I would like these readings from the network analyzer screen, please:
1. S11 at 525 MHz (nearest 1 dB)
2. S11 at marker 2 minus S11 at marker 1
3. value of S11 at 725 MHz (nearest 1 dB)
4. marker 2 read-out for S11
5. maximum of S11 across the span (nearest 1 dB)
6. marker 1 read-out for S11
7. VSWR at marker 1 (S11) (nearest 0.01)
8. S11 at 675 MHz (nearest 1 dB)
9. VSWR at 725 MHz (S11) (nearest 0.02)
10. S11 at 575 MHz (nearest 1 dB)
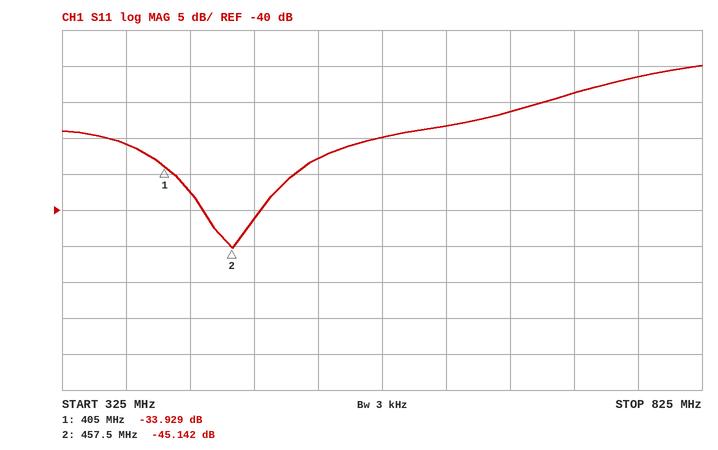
-33 dB
-11.213 dB
-24 dB
-45.142 dB
-20 dB
-33.929 dB
1.04
-26 dB
1.14
-30 dB
